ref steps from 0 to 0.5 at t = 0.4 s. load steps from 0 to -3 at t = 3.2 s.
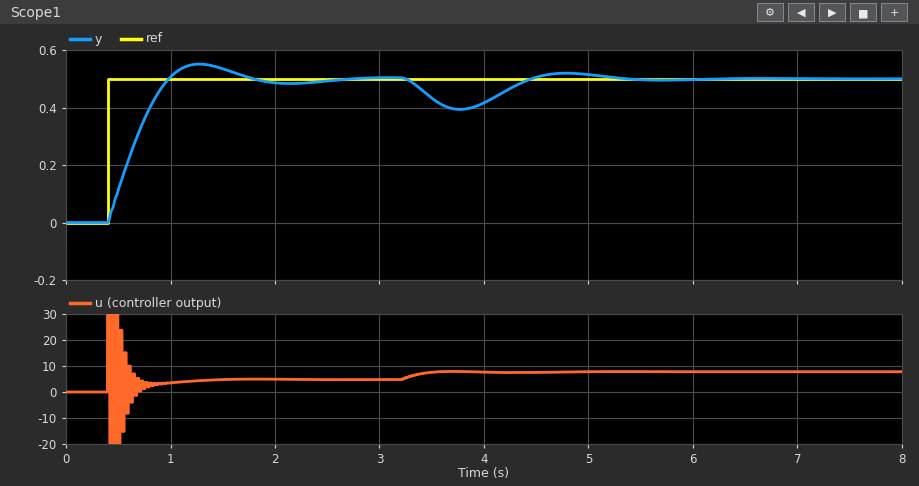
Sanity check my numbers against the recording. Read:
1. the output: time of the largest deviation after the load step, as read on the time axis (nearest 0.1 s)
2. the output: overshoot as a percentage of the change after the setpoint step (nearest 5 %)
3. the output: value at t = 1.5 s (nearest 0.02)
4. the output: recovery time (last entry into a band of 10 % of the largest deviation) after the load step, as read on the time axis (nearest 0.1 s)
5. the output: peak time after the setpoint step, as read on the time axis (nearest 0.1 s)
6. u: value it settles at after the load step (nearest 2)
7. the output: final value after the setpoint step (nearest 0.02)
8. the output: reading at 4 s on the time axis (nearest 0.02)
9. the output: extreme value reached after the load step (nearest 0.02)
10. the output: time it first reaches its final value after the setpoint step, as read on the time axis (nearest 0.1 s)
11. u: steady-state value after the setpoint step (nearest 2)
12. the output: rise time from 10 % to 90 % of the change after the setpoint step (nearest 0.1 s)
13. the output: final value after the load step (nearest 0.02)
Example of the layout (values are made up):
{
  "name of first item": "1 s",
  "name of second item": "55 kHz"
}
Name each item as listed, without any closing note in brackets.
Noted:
{
  "the output: time of the largest deviation after the load step, as read on the time axis": "3.8 s",
  "the output: overshoot as a percentage of the change after the setpoint step": "10 %",
  "the output: value at t = 1.5 s": "0.54",
  "the output: recovery time (last entry into a band of 10 % of the largest deviation) after the load step, as read on the time axis": "5.1 s",
  "the output: peak time after the setpoint step, as read on the time axis": "1.3 s",
  "u: value it settles at after the load step": "8",
  "the output: final value after the setpoint step": "0.50",
  "the output: reading at 4 s on the time axis": "0.42",
  "the output: extreme value reached after the load step": "0.40",
  "the output: time it first reaches its final value after the setpoint step, as read on the time axis": "1.0 s",
  "u: steady-state value after the setpoint step": "4",
  "the output: rise time from 10 % to 90 % of the change after the setpoint step": "0.4 s",
  "the output: final value after the load step": "0.50"
}
